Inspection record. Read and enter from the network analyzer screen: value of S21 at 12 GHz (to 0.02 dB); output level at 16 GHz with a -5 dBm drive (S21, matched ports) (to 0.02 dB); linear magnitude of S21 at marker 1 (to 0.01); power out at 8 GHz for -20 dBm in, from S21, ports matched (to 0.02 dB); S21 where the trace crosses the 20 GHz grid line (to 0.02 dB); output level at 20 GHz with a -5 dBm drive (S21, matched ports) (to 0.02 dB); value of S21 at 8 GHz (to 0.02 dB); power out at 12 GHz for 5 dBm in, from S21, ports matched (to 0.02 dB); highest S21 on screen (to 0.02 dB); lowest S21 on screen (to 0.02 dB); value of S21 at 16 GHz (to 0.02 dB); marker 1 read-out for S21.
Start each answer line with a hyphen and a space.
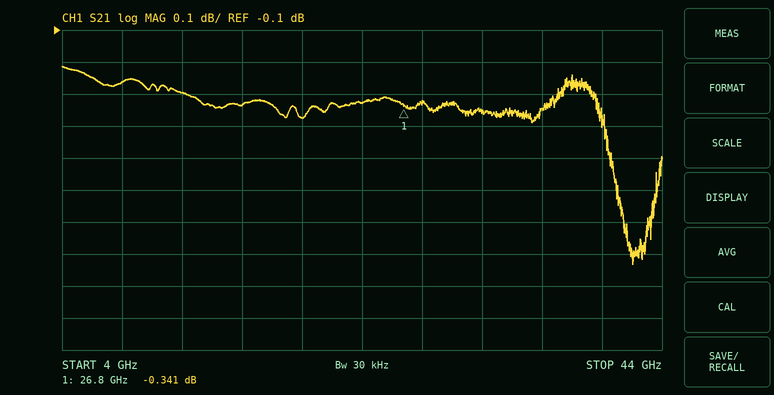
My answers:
- -0.30 dB
- -5.34 dBm
- 0.96
- -20.26 dBm
- -0.38 dB
- -5.38 dBm
- -0.26 dB
- 4.70 dBm
- -0.22 dB
- -0.84 dB
- -0.34 dB
- -0.341 dB
